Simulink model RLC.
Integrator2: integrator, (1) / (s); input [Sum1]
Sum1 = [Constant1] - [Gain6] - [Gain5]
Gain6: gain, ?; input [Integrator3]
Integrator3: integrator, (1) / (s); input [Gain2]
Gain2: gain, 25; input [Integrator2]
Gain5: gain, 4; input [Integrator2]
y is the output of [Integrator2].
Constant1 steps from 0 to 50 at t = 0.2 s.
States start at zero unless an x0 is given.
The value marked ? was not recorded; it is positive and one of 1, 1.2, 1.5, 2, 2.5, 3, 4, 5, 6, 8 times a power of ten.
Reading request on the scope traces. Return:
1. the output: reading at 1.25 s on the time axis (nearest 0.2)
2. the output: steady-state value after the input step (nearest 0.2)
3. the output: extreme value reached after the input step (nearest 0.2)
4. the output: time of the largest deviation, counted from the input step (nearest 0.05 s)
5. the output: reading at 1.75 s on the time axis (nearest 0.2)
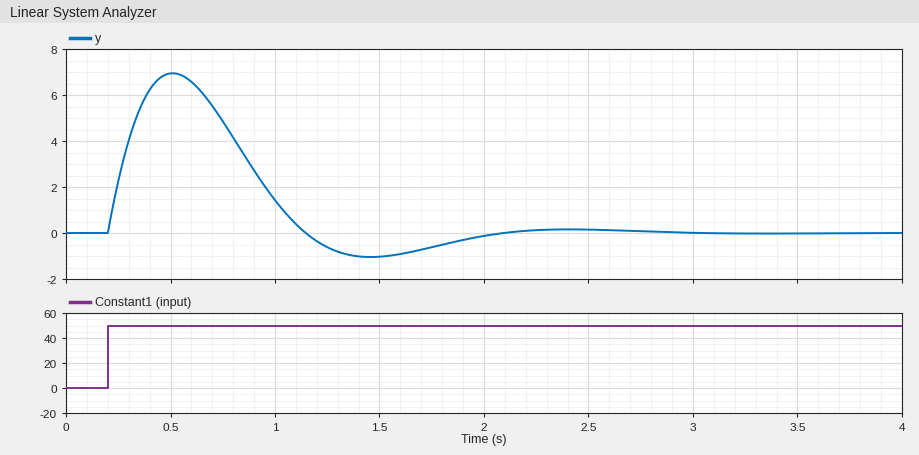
-0.6
0.0
7.0
0.30 s
-0.6
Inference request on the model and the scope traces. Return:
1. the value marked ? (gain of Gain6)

0.6
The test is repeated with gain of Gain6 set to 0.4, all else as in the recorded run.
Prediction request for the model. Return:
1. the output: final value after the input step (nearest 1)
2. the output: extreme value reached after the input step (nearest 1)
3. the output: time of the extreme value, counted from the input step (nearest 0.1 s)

0
8
0.4 s
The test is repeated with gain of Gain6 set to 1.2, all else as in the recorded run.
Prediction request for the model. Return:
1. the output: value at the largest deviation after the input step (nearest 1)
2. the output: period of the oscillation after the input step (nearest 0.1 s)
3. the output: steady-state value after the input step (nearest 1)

6
1.2 s
0
